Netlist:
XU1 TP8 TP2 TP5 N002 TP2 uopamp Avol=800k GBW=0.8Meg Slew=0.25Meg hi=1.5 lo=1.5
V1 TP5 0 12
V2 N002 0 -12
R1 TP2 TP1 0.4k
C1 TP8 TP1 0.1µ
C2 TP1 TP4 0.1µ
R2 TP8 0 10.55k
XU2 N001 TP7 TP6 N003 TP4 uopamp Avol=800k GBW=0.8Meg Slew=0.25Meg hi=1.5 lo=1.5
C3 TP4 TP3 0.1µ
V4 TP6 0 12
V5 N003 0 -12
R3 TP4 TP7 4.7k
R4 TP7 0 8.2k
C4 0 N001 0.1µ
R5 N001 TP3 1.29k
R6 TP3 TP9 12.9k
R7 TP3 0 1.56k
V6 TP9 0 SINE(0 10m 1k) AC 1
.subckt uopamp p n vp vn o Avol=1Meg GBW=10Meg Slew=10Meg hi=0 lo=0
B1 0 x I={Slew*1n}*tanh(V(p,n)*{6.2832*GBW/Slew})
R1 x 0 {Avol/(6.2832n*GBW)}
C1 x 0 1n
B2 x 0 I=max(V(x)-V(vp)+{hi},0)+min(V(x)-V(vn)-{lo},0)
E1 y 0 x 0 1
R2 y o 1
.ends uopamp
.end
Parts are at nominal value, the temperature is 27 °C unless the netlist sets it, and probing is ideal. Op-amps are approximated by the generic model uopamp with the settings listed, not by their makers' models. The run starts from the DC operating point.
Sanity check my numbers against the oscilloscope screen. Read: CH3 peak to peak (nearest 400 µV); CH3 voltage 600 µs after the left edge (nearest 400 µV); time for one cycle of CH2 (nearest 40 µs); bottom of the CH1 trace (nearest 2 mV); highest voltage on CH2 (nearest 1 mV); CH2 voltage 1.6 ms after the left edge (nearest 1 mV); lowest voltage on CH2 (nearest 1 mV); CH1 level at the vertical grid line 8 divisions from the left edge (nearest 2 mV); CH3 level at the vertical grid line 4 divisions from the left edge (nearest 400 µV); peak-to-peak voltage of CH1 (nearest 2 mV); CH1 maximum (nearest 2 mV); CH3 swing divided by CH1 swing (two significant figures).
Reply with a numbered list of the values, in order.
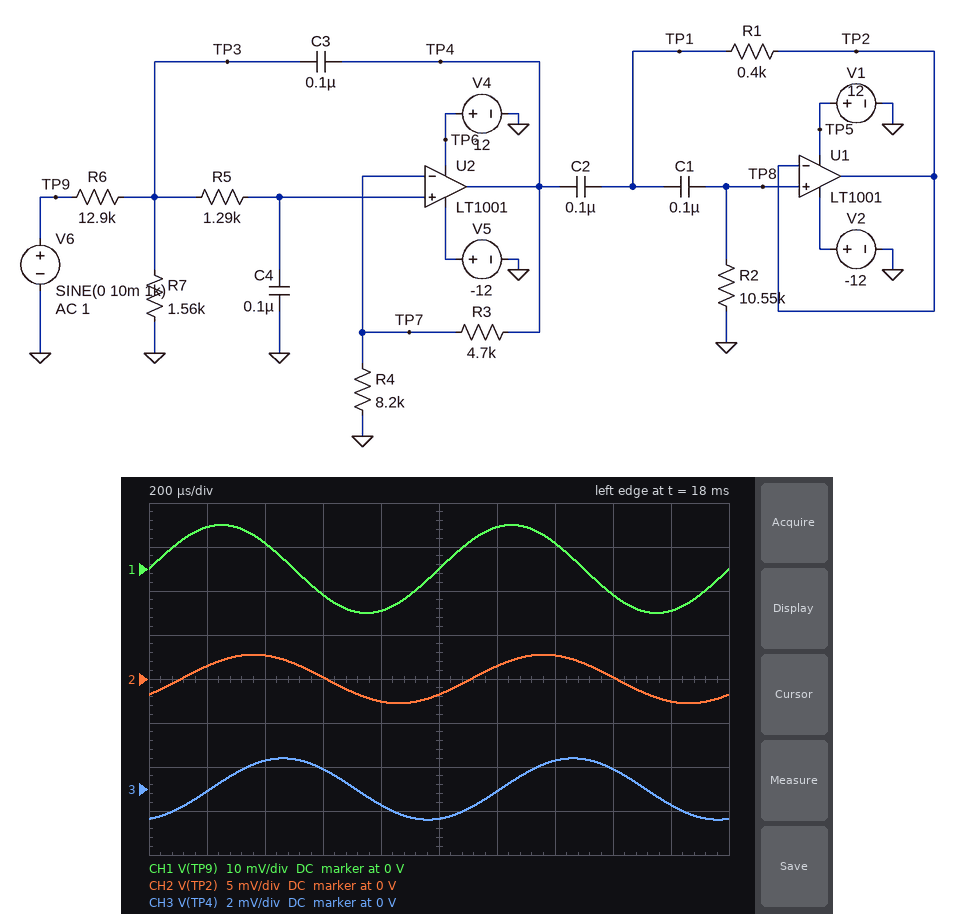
1. 2.8 mV
2. 800 µV
3. 1.00 ms
4. -10 mV
5. 3 mV
6. 0 V
7. -3 mV
8. -6 mV
9. -800 µV
10. 20 mV
11. 10 mV
12. 0.14
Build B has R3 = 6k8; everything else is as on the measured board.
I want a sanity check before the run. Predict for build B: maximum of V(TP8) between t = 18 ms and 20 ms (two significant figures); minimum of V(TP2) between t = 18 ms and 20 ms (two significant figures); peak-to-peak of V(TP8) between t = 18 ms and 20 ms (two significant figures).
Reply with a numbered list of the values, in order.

1. 3.9 mV
2. -3.9 mV
3. 7.8 mV
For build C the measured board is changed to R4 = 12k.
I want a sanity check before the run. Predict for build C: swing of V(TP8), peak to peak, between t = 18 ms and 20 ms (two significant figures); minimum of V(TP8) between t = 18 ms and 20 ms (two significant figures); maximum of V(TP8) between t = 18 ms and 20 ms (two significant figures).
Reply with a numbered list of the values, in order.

1. 4.3 mV
2. -2.2 mV
3. 2.2 mV
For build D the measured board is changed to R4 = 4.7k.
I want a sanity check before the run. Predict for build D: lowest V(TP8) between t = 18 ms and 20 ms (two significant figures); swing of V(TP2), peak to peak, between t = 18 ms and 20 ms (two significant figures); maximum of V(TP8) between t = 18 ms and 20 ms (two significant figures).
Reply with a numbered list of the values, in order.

1. -5.0 mV
2. 9.9 mV
3. 5.0 mV
